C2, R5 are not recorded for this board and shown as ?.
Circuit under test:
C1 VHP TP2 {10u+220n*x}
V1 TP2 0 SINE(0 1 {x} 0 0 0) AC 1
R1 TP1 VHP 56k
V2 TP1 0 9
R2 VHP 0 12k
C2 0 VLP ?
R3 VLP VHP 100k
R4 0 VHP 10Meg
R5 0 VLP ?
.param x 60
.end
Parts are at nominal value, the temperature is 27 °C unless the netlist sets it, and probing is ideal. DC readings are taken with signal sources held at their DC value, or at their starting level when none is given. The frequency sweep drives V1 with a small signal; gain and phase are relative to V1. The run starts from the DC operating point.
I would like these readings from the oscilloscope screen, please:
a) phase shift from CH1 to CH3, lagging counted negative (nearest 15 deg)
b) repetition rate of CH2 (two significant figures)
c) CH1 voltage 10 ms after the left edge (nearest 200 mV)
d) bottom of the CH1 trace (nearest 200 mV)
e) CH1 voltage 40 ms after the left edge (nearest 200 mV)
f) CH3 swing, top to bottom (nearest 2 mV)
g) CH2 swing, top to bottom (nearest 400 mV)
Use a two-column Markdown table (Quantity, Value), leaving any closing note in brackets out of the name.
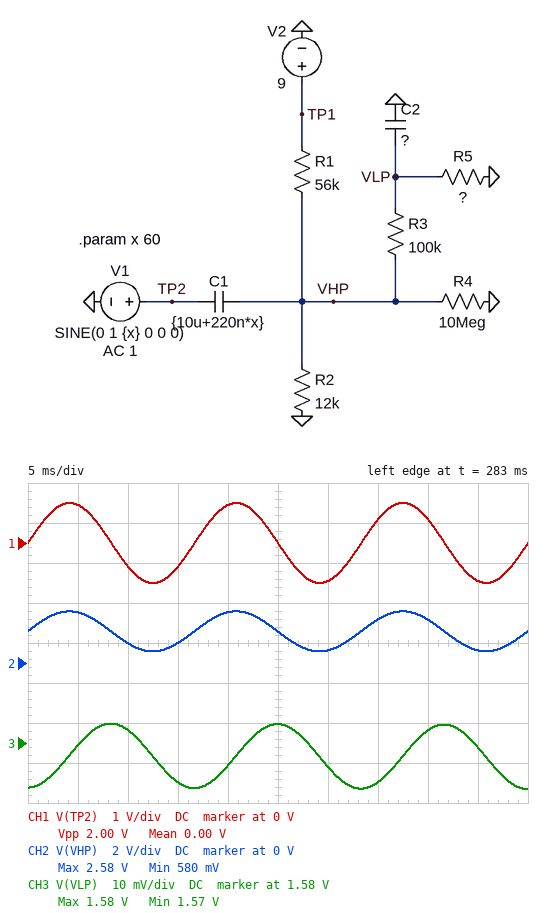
| Quantity | Value |
|---|---|
| phase shift from CH1 to CH3, lagging counted negative | -90 deg |
| repetition rate of CH2 | 60 Hz |
| CH1 voltage 10 ms after the left edge | -600 mV |
| bottom of the CH1 trace | -1.0 V |
| CH1 voltage 40 ms after the left edge | 600 mV |
| CH3 swing, top to bottom | 16 mV |
| CH2 swing, top to bottom | 2.0 V |
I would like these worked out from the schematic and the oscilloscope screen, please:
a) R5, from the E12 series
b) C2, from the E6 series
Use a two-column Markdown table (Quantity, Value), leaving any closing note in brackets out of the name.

| Quantity | Value |
|---|---|
| R5, from the E12 series | 18 MΩ |
| C2, from the E6 series | 3.3 µF |
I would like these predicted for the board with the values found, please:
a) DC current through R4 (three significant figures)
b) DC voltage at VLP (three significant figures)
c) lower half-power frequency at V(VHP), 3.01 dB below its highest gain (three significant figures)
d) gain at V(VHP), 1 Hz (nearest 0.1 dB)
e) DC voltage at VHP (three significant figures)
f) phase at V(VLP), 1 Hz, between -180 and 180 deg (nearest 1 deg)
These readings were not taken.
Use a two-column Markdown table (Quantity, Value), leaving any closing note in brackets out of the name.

| Quantity | Value |
|---|---|
| DC current through R4 | 159 nA |
| DC voltage at VLP | 1.58 V |
| lower half-power frequency at V(VHP), 3.01 dB below its highest gain | 776 mHz |
| gain at V(VHP), 1 Hz | -2.1 dB |
| DC voltage at VHP | 1.59 V |
| phase at V(VLP), 1 Hz, between -180 and 180 deg | -28 deg |
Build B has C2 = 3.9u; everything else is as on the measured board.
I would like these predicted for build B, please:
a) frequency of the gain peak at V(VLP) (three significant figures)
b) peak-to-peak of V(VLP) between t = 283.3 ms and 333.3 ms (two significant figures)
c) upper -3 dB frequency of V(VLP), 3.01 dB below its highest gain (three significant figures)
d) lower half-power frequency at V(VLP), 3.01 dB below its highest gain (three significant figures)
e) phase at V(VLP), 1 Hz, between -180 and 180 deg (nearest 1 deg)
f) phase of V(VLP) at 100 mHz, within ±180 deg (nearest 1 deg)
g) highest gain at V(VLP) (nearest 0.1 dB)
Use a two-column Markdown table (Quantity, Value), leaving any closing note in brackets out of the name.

| Quantity | Value |
|---|---|
| frequency of the gain peak at V(VLP) | 534 mHz |
| peak-to-peak of V(VLP) between t = 283.3 ms and 333.3 ms | 14 mV |
| upper -3 dB frequency of V(VLP), 3.01 dB below its highest gain | 1.38 Hz |
| lower half-power frequency at V(VLP), 3.01 dB below its highest gain | 207 mHz |
| phase at V(VLP), 1 Hz, between -180 and 180 deg | -31 deg |
| phase of V(VLP) at 100 mHz, within ±180 deg | 67 deg |
| highest gain at V(VLP) | -9.2 dB |
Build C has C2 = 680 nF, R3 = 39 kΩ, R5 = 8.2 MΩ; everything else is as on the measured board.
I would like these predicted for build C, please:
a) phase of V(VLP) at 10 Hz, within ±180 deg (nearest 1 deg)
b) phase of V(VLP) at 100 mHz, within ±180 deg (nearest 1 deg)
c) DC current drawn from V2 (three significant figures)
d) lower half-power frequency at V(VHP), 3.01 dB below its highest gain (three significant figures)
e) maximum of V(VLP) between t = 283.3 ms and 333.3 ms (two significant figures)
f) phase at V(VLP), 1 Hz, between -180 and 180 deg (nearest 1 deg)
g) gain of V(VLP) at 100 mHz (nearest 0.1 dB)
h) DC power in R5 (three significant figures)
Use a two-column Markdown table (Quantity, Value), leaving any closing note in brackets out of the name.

| Quantity | Value |
|---|---|
| phase of V(VLP) at 10 Hz, within ±180 deg | -54 deg |
| phase of V(VLP) at 100 mHz, within ±180 deg | 81 deg |
| DC current drawn from V2 | 132 µA |
| lower half-power frequency at V(VHP), 3.01 dB below its highest gain | 719 mHz |
| maximum of V(VLP) between t = 283.3 ms and 333.3 ms | 1.7 V |
| phase at V(VLP), 1 Hz, between -180 and 180 deg | 25 deg |
| gain of V(VLP) at 100 mHz | -17.0 dB |
| DC power in R5 | 303 nW |
